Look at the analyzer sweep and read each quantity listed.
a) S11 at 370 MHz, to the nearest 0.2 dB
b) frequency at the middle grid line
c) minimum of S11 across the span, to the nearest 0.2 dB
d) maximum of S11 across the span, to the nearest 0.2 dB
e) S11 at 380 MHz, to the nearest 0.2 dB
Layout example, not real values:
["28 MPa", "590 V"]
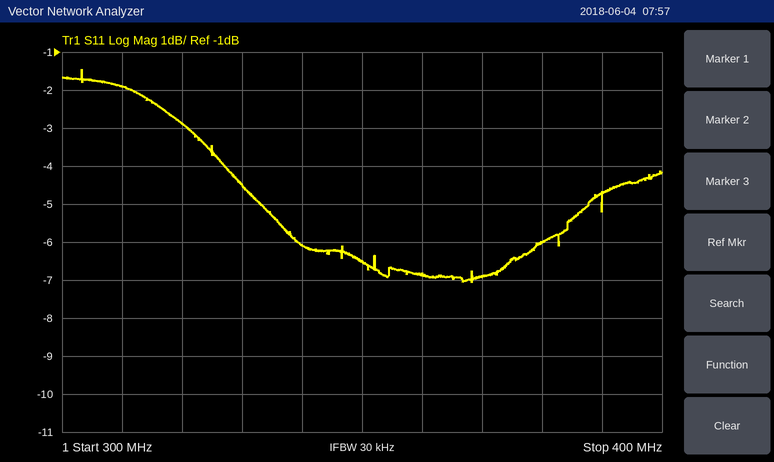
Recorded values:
["-7.0 dB", "350 MHz", "-7.0 dB", "-1.4 dB", "-6.0 dB"]
